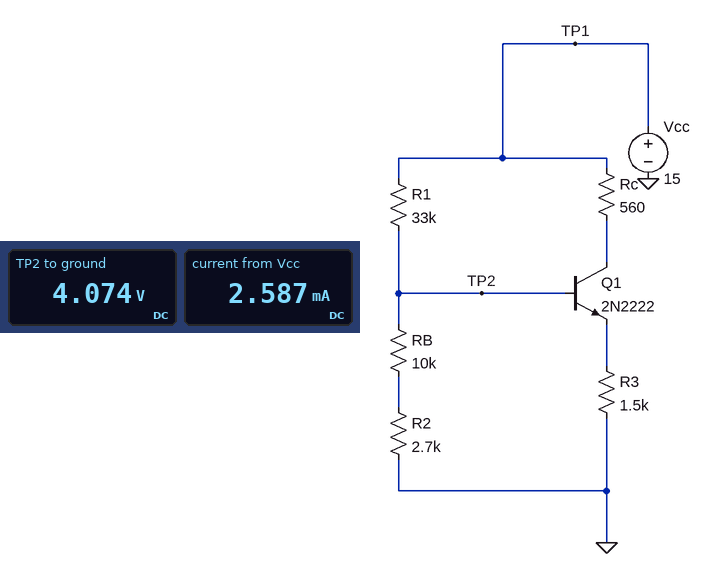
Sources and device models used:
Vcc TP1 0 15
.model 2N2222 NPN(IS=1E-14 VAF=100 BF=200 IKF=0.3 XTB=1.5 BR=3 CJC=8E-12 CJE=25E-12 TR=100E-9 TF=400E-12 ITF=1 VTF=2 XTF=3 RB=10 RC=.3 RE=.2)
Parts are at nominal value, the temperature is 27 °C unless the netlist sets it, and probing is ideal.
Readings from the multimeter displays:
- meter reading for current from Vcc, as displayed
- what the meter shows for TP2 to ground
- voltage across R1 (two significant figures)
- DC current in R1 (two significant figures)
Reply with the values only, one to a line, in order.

2.587 mA
4.074 V
11 V
330 µA
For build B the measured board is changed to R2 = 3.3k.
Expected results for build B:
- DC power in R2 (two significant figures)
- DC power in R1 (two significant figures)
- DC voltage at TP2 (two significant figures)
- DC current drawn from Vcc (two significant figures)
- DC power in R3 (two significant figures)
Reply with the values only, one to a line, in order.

330 µW
3.5 mW
4.2 V
2.7 mA
8.3 mW
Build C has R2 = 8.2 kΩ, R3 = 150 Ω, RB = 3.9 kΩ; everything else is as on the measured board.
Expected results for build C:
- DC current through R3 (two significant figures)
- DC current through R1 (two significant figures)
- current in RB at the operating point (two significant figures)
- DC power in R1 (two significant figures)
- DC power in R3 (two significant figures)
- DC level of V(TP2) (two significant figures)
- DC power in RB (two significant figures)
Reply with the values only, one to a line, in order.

17 mA
360 µA
270 µA
4.2 mW
43 mW
3.3 V
280 µW
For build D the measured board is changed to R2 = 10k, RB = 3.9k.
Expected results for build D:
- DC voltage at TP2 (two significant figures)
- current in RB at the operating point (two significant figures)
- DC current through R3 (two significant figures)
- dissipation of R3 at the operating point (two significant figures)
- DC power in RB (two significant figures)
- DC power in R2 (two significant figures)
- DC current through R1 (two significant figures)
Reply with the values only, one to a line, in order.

4.3 V
310 µA
2.4 mA
8.9 mW
380 µW
970 µW
320 µA
